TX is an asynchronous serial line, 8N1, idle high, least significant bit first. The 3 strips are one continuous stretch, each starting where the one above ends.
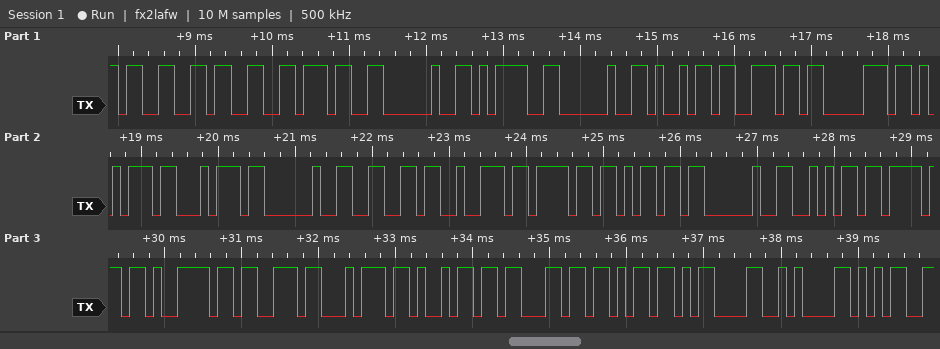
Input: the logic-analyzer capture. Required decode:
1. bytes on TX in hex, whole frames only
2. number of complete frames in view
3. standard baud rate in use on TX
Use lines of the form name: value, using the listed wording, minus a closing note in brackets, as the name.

bytes on TX in hex, whole frames only: 33 33 37 20 3D 20 69 6E 70 75 74 20 66 72 6F 6D 20 6A 6F 79 73 74 69 63 6B 0D 0A 35
number of complete frames in view: 28
standard baud rate in use on TX: 9600 baud
